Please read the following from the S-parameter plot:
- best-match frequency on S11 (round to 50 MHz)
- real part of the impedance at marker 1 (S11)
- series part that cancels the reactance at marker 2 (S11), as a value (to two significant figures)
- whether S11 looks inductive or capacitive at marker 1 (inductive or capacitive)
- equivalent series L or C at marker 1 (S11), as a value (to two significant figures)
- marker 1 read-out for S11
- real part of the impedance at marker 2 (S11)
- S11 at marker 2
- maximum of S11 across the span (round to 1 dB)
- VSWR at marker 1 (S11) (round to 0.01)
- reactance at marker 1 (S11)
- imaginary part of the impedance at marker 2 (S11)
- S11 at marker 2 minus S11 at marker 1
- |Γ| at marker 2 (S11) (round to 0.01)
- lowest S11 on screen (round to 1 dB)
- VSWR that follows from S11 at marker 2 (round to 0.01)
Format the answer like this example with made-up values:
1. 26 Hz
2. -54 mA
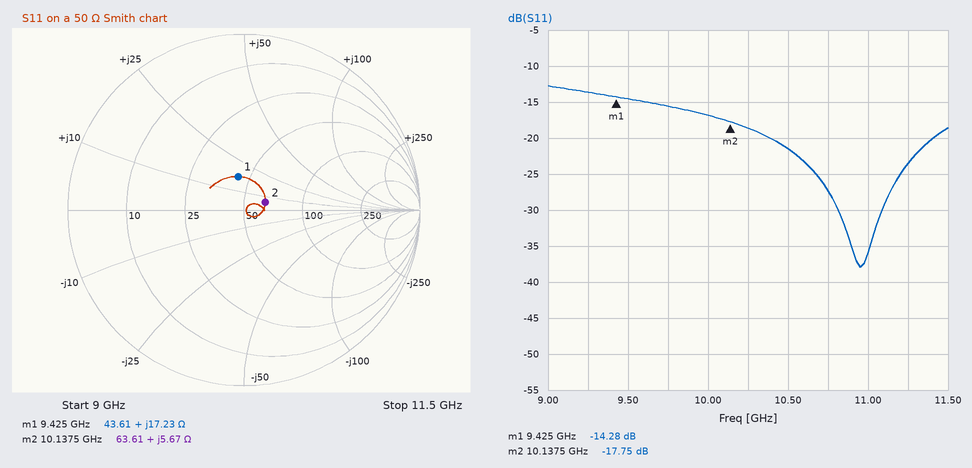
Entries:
1. 10.95 GHz
2. 43.61 Ω
3. 2.8 pF
4. inductive
5. 290 pH
6. -14.28 dB
7. 63.61 Ω
8. -17.75 dB
9. -13 dB
10. 1.48
11. +17.23 Ω
12. +5.67 Ω
13. -3.47 dB
14. 0.13
15. -38 dB
16. 1.30
